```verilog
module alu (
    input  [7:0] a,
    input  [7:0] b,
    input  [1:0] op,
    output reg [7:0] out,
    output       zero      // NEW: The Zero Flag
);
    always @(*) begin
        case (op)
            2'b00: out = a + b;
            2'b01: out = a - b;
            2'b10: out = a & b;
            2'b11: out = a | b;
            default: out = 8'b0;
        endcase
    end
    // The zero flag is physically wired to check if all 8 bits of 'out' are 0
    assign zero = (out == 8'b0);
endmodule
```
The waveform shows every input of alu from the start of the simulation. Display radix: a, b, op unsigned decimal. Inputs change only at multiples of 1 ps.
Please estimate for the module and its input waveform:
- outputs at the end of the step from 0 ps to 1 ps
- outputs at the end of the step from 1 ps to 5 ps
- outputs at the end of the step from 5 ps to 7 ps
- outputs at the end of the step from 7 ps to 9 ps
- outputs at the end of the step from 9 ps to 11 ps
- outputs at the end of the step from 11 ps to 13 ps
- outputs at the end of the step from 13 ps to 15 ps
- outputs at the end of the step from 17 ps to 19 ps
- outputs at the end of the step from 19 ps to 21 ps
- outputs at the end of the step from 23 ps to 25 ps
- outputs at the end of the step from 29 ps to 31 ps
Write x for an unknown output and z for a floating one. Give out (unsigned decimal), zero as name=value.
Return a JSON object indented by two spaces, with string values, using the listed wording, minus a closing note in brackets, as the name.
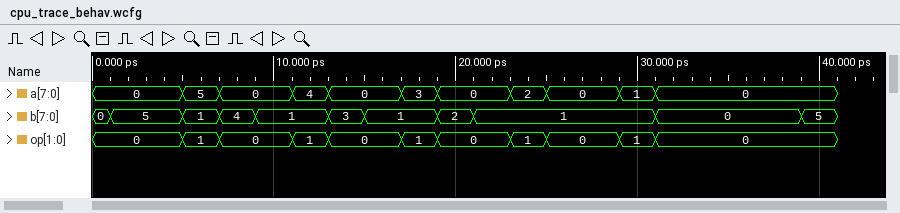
{
  "outputs at the end of the step from 0 ps to 1 ps": "out=0, zero=1",
  "outputs at the end of the step from 1 ps to 5 ps": "out=5, zero=0",
  "outputs at the end of the step from 5 ps to 7 ps": "out=4, zero=0",
  "outputs at the end of the step from 7 ps to 9 ps": "out=4, zero=0",
  "outputs at the end of the step from 9 ps to 11 ps": "out=1, zero=0",
  "outputs at the end of the step from 11 ps to 13 ps": "out=3, zero=0",
  "outputs at the end of the step from 13 ps to 15 ps": "out=3, zero=0",
  "outputs at the end of the step from 17 ps to 19 ps": "out=2, zero=0",
  "outputs at the end of the step from 19 ps to 21 ps": "out=2, zero=0",
  "outputs at the end of the step from 23 ps to 25 ps": "out=1, zero=0",
  "outputs at the end of the step from 29 ps to 31 ps": "out=0, zero=1"
}
